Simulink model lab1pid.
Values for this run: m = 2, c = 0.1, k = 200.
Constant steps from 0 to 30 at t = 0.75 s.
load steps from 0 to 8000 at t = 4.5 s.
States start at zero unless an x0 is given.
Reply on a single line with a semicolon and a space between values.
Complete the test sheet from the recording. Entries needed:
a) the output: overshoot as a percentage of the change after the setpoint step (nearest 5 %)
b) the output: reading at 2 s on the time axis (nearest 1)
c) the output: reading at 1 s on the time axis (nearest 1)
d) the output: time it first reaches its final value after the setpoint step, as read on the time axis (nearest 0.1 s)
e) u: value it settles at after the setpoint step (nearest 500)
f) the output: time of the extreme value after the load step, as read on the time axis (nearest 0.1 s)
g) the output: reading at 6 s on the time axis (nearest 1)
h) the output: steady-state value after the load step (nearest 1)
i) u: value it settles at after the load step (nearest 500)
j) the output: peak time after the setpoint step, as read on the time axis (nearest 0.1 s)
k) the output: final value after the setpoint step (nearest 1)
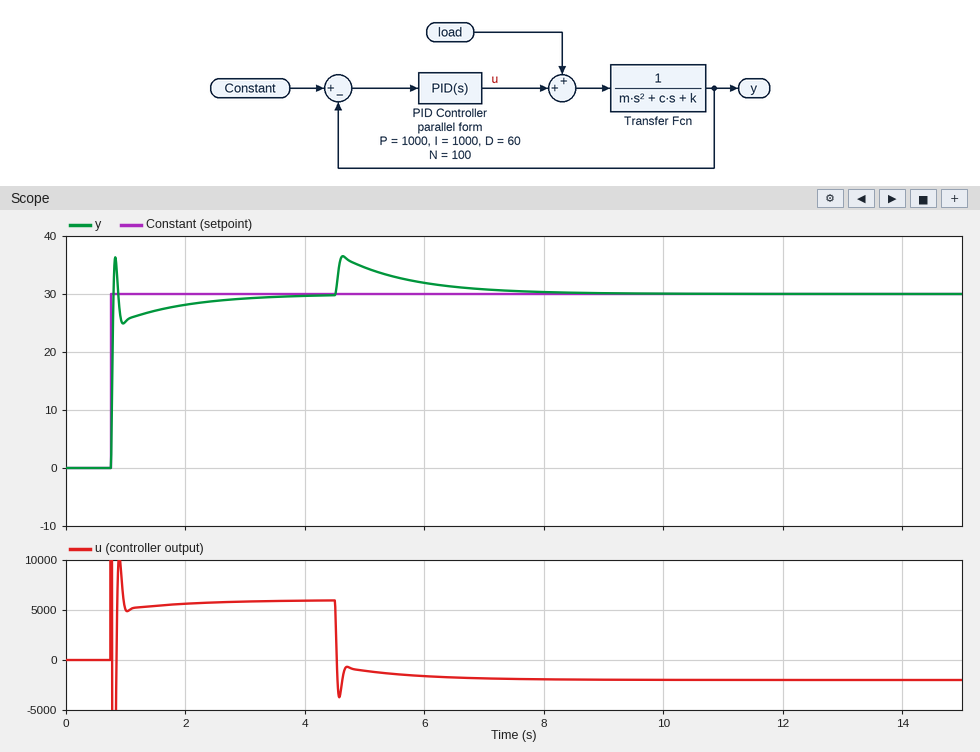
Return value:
20 %; 28; 25; 0.8 s; 6000; 4.6 s; 32; 30; -2000; 0.8 s; 30
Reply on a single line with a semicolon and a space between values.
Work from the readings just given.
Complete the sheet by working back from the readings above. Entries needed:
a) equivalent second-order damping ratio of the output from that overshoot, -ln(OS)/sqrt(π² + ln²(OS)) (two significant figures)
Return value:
0.46
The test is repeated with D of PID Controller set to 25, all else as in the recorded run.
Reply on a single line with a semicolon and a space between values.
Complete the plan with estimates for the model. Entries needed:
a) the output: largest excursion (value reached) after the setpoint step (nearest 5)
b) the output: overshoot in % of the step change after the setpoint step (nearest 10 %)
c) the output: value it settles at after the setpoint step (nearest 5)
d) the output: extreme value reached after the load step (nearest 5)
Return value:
40; 40 %; 30; 40
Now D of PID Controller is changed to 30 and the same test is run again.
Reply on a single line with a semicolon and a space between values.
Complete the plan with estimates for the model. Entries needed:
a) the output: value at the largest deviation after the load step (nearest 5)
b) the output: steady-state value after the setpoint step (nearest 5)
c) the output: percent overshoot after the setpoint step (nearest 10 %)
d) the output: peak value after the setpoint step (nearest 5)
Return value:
40; 30; 30 %; 40
